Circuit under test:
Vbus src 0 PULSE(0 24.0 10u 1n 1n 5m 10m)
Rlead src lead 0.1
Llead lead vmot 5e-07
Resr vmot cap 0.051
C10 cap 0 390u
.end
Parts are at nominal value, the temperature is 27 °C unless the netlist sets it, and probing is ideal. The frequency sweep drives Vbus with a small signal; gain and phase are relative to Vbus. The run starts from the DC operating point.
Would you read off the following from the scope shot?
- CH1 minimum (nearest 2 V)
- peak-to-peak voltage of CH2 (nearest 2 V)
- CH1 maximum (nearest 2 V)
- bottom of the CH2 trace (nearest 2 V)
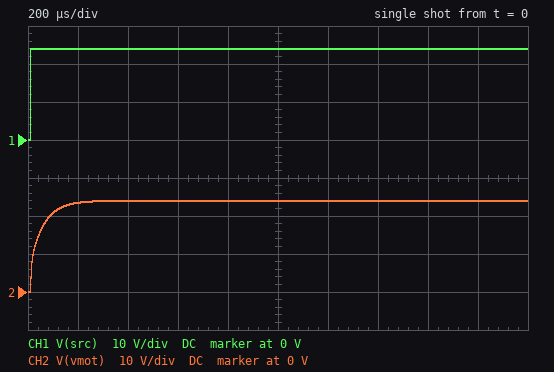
0 V
24 V
24 V
0 V
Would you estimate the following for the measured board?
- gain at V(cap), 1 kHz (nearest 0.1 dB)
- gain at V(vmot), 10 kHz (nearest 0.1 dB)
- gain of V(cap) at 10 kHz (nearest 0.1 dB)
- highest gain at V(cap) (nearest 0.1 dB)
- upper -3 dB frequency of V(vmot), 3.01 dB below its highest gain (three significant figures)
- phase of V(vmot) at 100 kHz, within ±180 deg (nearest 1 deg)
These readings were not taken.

-0.5 dB
-7.3 dB
-11.4 dB
0 dB
3.32 kHz
-69 deg
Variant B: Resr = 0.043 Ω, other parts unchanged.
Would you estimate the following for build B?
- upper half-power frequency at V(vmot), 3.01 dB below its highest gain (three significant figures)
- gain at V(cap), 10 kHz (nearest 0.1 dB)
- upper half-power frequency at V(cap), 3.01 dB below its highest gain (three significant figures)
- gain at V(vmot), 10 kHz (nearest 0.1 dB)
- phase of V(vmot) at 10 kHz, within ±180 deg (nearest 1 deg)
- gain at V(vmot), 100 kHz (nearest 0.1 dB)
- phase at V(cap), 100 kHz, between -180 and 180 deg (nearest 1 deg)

3.41 kHz
-10.9 dB
3.04 kHz
-7.7 dB
-40 deg
-18.0 dB
-155 deg
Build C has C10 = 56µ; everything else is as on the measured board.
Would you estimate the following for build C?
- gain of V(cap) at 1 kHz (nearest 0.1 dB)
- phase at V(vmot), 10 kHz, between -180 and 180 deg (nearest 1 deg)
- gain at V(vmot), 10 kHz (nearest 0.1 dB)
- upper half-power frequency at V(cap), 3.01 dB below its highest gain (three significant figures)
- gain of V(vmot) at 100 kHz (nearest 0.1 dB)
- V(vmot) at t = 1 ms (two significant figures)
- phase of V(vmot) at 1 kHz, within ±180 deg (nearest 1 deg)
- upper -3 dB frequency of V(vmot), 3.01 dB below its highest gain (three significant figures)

0 dB
-21 deg
-0.2 dB
26.2 kHz
-14.9 dB
24 V
-2 deg
30.3 kHz
